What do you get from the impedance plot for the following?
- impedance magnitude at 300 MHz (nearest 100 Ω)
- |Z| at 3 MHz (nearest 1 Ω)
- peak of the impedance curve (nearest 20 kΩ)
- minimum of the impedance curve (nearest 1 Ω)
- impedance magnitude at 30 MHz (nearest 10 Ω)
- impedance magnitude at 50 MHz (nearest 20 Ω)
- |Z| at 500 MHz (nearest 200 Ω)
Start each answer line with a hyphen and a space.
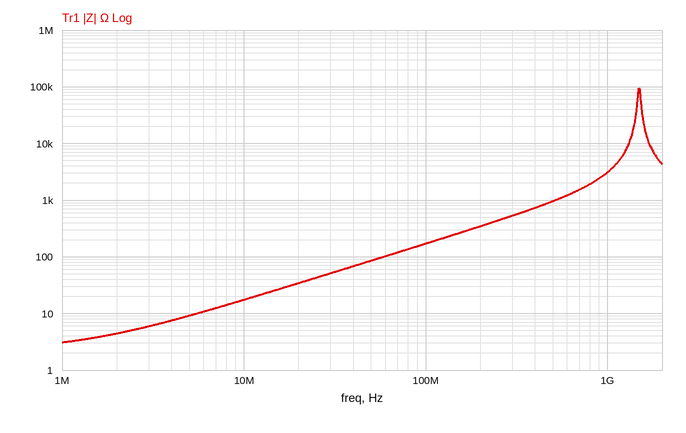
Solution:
- 500 Ω
- 6 Ω
- 100 kΩ
- 3 Ω
- 50 Ω
- 80 Ω
- 1.0 kΩ
